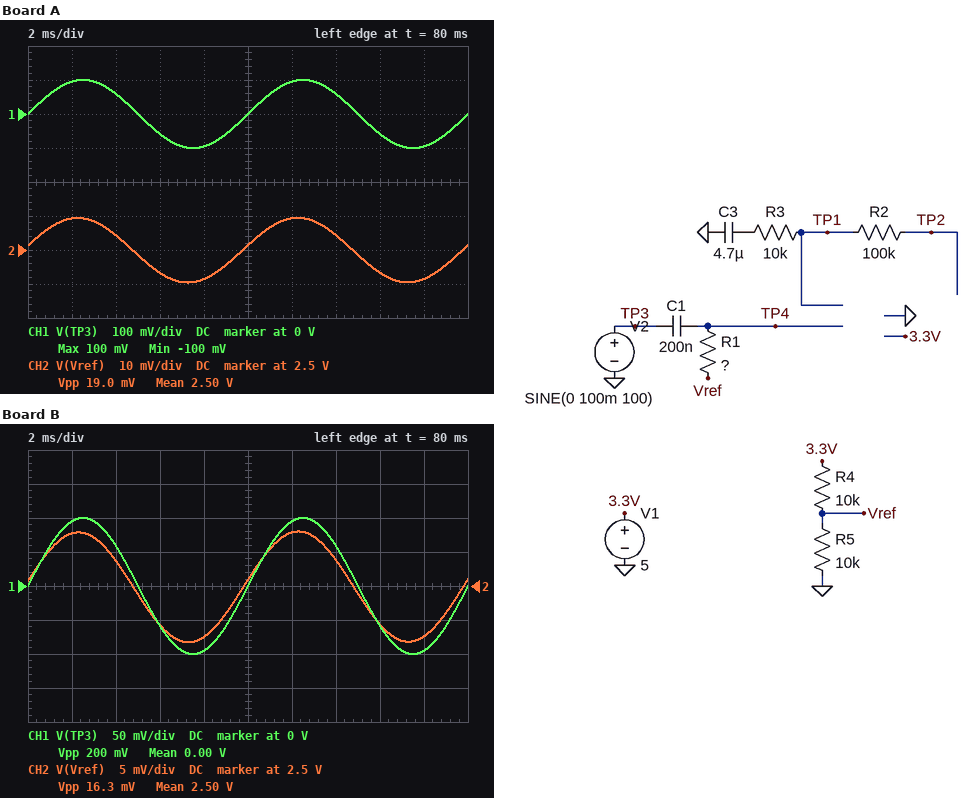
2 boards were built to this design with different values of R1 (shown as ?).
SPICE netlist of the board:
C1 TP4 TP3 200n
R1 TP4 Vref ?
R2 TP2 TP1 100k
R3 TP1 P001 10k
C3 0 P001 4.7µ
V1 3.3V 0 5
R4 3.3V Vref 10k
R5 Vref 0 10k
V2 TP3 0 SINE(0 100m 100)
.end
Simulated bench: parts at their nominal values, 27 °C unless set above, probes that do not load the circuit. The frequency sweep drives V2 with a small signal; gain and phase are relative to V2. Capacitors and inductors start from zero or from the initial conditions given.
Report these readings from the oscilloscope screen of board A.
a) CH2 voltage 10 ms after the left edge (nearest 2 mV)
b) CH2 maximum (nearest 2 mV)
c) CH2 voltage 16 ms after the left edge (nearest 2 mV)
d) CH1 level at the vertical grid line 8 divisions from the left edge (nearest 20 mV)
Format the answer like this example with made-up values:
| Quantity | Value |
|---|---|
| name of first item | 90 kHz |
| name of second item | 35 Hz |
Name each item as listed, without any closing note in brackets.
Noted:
| Quantity | Value |
|---|---|
| CH2 voltage 10 ms after the left edge | 2.502 V |
| CH2 maximum | 2.510 V |
| CH2 voltage 16 ms after the left edge | 2.494 V |
| CH1 level at the vertical grid line 8 divisions from the left edge | -60 mV |
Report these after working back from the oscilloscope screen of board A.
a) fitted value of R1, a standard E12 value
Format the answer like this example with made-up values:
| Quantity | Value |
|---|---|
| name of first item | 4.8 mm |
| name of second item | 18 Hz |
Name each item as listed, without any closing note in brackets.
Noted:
| Quantity | Value |
|---|---|
| fitted value of R1, a standard E12 value | 47 kΩ |
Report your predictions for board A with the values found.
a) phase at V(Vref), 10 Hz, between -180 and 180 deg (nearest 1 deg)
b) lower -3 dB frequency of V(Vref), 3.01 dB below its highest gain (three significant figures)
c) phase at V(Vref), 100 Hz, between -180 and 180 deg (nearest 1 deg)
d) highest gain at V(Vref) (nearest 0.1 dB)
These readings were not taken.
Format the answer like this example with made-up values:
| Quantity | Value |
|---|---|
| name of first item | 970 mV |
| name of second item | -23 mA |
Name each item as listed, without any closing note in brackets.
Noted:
| Quantity | Value |
|---|---|
| phase at V(Vref), 10 Hz, between -180 and 180 deg | 57 deg |
| lower -3 dB frequency of V(Vref), 3.01 dB below its highest gain | 15.3 Hz |
| phase at V(Vref), 100 Hz, between -180 and 180 deg | 9 deg |
| highest gain at V(Vref) | -20.3 dB |
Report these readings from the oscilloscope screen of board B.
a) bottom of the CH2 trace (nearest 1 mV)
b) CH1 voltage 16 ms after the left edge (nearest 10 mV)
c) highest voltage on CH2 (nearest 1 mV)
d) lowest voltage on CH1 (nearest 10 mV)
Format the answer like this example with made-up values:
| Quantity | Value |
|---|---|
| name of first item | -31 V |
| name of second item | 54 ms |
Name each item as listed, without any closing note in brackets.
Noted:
| Quantity | Value |
|---|---|
| bottom of the CH2 trace | 2.492 V |
| CH1 voltage 16 ms after the left edge | -60 mV |
| highest voltage on CH2 | 2.508 V |
| lowest voltage on CH1 | -100 mV |
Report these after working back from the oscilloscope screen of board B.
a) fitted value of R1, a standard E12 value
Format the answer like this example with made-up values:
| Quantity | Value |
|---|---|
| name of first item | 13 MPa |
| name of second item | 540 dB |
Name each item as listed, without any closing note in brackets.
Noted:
| Quantity | Value |
|---|---|
| fitted value of R1, a standard E12 value | 56 kΩ |
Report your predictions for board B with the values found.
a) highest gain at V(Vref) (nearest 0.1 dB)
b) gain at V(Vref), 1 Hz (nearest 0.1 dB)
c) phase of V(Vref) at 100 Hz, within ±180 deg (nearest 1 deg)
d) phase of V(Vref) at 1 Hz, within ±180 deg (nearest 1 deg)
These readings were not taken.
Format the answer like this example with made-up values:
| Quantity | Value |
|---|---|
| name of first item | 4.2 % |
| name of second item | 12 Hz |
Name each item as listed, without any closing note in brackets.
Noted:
| Quantity | Value |
|---|---|
| highest gain at V(Vref) | -21.7 dB |
| gain at V(Vref), 1 Hz | -44.1 dB |
| phase of V(Vref) at 100 Hz, within ±180 deg | 7 deg |
| phase of V(Vref) at 1 Hz, within ±180 deg | 86 deg |
